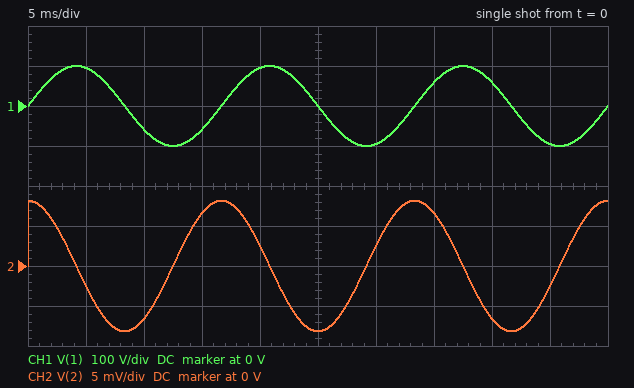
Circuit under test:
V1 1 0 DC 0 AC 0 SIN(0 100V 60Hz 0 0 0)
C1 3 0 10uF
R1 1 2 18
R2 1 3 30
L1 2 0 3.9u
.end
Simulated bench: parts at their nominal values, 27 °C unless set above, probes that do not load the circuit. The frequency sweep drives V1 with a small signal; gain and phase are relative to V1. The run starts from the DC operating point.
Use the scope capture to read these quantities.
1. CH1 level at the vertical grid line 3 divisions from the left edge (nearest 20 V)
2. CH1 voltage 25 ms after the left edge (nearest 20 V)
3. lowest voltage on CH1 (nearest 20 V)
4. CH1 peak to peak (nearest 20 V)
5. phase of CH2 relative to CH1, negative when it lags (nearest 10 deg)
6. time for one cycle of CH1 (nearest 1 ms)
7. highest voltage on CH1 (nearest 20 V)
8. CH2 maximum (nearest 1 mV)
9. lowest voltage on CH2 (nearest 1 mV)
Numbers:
-60 V
0 V
-100 V
200 V
90 deg
17 ms
100 V
8 mV
-8 mV
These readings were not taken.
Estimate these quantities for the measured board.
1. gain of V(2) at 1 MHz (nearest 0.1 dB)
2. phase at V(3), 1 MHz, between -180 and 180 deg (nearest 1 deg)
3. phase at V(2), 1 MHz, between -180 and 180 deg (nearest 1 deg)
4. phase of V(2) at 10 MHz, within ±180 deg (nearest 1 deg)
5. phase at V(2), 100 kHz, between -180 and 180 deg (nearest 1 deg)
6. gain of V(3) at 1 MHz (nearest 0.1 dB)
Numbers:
-1.9 dB
-90 deg
36 deg
4 deg
82 deg
-65.5 dB
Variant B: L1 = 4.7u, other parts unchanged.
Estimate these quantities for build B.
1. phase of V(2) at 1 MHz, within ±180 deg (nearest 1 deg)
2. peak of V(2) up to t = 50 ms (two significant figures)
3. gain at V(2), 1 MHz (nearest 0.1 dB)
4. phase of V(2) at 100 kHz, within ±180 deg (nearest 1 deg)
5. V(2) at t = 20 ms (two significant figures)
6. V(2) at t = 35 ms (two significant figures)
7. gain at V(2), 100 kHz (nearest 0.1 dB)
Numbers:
31 deg
9.9 mV
-1.4 dB
81 deg
3.0 mV
8.0 mV
-15.8 dB
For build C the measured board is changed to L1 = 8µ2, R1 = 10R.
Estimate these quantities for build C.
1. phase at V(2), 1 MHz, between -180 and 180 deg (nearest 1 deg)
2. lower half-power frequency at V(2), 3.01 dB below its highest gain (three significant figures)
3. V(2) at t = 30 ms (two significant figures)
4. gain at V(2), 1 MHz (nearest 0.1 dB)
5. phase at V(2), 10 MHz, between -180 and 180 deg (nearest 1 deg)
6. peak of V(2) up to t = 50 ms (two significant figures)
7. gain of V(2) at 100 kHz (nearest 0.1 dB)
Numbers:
11 deg
194 kHz
9.5 mV
-0.2 dB
1 deg
31 mV
-6.8 dB
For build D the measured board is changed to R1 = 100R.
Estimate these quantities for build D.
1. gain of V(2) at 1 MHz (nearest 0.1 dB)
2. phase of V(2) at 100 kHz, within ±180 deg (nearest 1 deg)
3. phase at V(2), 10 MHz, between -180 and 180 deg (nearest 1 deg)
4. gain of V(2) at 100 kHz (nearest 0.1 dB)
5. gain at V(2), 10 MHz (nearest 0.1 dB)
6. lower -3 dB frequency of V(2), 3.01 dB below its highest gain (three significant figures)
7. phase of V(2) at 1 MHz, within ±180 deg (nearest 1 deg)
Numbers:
-12.5 dB
89 deg
22 deg
-32.2 dB
-0.7 dB
4.08 MHz
76 deg
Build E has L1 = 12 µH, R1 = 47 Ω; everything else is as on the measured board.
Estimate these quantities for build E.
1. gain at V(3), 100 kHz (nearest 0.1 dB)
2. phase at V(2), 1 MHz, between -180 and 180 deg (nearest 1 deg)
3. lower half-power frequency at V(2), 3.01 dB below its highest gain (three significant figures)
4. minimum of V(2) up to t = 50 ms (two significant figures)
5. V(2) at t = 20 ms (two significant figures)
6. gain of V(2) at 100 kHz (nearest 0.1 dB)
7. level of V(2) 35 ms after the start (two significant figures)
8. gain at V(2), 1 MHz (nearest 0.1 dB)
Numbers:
-45.5 dB
32 deg
623 kHz
-9.6 mV
3.0 mV
-16.0 dB
7.8 mV
-1.4 dB
